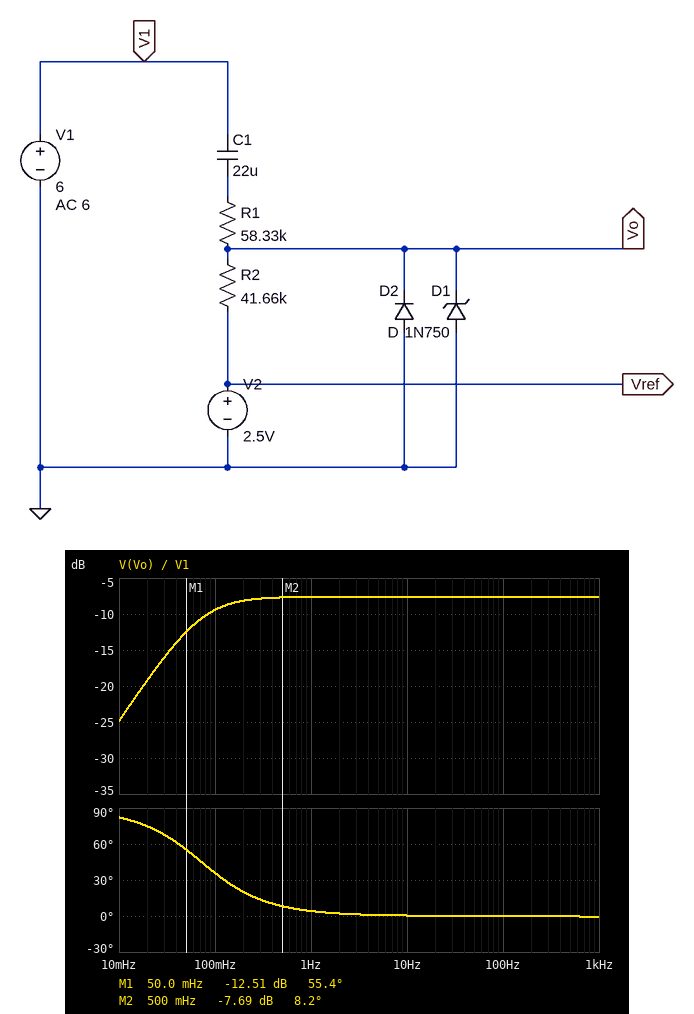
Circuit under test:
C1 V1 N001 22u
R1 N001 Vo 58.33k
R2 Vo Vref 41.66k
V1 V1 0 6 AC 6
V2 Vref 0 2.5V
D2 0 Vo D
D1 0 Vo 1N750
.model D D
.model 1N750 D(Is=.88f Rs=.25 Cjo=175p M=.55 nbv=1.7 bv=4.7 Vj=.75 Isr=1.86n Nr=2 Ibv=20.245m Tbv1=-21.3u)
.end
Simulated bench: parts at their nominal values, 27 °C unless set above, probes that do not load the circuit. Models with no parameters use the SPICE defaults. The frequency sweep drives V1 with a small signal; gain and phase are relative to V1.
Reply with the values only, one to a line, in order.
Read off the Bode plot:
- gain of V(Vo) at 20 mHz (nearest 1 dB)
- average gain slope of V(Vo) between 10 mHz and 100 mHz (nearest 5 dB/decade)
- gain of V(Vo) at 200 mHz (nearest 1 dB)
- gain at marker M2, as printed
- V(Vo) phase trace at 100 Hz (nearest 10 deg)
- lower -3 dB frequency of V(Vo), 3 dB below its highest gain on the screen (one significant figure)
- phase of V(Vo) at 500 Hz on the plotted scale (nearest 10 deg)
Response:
-19 dB
15 dB/decade
-8 dB
-7.69 dB
0 deg
70 mHz
0 deg
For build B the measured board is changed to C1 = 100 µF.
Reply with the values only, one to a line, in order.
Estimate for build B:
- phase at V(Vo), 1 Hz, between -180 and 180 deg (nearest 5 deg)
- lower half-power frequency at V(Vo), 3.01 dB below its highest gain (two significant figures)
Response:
0 deg
16 mHz
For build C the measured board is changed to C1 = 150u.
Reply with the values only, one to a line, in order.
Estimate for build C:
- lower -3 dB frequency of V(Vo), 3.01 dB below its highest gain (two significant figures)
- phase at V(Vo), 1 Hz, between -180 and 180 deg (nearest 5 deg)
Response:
11 mHz
0 deg
